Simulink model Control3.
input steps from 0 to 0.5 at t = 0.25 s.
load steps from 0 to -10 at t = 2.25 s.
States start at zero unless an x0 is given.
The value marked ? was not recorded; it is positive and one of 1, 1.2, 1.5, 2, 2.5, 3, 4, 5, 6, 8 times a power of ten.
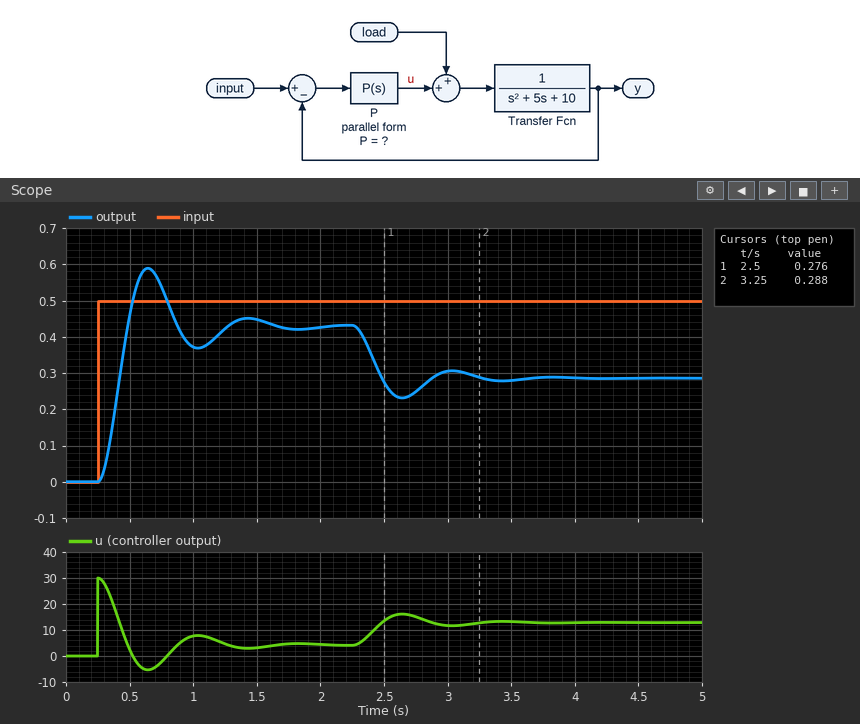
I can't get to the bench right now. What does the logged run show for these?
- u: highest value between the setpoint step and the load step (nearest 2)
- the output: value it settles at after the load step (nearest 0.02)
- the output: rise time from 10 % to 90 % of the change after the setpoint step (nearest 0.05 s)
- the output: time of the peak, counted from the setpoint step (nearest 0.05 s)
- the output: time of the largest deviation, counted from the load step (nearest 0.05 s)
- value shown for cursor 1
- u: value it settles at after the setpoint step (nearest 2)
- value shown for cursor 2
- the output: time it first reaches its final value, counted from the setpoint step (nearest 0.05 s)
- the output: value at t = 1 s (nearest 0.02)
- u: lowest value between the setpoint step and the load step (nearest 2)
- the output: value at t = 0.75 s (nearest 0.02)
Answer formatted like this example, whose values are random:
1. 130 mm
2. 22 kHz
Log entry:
1. 30
2. 0.28
3. 0.15 s
4. 0.40 s
5. 0.40 s
6. 0.276
7. 4
8. 0.288
9. 0.25 s
10. 0.38
11. -6
12. 0.54
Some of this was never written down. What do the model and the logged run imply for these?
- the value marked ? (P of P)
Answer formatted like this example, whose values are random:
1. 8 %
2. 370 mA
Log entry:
1. 60
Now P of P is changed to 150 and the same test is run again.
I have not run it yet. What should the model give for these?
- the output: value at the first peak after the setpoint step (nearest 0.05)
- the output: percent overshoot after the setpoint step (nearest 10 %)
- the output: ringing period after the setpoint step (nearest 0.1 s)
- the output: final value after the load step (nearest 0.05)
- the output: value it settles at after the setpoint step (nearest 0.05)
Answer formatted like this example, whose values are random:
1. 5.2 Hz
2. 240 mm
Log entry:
1. 0.70
2. 50 %
3. 0.5 s
4. 0.40
5. 0.45
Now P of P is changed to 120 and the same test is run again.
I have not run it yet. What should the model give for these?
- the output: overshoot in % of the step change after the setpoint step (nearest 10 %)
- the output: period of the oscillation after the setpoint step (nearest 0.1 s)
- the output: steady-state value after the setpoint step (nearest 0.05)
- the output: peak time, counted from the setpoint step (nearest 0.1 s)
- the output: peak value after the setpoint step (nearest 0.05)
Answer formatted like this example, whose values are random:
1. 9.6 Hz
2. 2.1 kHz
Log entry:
1. 50 %
2. 0.6 s
3. 0.45
4. 0.3 s
5. 0.70
